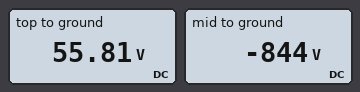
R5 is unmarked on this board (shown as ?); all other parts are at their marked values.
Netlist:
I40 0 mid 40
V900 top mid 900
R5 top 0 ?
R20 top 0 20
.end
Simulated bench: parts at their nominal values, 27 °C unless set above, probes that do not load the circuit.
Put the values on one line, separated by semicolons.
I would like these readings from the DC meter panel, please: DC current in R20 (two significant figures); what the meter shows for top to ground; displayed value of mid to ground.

2.8 A; 55.81 V; -844 V
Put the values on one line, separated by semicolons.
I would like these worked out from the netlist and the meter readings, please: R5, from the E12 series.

1.5 Ω
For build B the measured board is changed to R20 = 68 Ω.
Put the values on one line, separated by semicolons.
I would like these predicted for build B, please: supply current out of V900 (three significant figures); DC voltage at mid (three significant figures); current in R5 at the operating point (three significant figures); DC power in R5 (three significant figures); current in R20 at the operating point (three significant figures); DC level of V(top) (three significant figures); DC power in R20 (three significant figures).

40.0 A; -841 V; 39.1 A; 2.30 kW; 863 mA; 58.7 V; 50.7 W
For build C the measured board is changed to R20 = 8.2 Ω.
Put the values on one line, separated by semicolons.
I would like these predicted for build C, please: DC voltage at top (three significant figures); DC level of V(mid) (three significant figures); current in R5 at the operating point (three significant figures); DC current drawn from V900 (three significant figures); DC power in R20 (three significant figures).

50.7 V; -849 V; 33.8 A; 40.0 A; 314 W
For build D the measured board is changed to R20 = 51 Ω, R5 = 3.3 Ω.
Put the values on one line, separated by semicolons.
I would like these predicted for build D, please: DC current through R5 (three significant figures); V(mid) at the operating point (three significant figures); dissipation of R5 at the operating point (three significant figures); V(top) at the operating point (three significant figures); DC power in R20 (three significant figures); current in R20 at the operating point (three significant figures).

37.6 A; -776 V; 4.66 kW; 124 V; 301 W; 2.43 A
